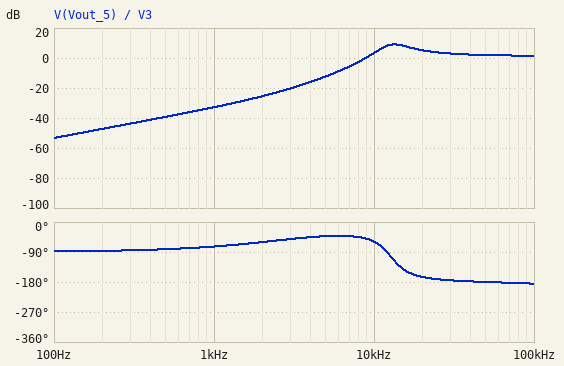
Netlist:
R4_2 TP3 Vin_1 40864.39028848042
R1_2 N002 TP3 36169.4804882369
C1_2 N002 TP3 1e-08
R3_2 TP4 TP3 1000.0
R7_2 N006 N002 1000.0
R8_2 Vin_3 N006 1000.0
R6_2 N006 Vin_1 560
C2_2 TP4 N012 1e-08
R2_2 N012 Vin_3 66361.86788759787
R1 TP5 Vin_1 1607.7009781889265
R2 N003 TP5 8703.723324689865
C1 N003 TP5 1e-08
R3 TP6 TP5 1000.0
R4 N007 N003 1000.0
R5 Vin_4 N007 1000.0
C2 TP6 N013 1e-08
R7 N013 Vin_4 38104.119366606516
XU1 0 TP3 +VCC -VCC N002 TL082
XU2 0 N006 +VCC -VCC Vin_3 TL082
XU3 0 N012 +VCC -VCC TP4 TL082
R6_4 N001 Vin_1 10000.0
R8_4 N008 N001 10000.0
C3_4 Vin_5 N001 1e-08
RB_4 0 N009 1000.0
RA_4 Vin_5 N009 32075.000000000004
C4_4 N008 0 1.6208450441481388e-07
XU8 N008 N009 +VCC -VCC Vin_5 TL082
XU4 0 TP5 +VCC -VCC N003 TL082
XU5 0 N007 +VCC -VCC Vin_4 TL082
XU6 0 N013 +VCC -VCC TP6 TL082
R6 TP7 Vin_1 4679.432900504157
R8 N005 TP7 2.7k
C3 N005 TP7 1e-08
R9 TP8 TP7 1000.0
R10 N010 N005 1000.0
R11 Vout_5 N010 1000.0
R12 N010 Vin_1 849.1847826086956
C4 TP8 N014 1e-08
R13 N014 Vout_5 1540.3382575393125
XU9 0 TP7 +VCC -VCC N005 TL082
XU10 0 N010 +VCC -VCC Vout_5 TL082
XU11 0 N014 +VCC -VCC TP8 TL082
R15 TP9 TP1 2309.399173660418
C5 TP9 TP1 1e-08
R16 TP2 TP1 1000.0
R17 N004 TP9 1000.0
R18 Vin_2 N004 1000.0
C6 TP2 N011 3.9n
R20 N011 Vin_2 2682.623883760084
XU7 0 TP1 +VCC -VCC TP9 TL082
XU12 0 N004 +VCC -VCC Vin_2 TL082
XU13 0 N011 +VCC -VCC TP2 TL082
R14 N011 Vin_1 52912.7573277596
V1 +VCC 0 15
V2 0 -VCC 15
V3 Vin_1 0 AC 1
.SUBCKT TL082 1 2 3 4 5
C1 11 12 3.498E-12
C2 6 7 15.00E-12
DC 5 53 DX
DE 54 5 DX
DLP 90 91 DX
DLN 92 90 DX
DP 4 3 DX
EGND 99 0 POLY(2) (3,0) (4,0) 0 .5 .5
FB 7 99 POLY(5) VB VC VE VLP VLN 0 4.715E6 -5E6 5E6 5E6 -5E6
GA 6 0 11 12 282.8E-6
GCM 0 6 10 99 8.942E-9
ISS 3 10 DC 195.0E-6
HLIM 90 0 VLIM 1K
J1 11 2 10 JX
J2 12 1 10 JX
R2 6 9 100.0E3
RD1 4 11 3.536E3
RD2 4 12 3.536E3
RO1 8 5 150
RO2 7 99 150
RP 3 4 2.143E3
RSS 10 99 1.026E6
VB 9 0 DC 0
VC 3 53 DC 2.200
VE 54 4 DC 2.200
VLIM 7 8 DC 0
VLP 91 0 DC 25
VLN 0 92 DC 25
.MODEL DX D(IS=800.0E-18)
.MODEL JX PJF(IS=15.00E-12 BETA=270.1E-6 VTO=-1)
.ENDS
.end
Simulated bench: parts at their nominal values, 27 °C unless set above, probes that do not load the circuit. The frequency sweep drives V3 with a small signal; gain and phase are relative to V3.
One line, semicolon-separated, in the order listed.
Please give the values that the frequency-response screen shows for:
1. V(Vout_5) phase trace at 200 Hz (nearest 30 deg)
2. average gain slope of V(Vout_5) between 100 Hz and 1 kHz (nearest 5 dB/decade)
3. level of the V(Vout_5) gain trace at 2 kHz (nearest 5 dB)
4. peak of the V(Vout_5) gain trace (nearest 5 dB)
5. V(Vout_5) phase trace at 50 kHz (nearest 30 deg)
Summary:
-90 deg; 20 dB/decade; -25 dB; 10 dB; -180 deg
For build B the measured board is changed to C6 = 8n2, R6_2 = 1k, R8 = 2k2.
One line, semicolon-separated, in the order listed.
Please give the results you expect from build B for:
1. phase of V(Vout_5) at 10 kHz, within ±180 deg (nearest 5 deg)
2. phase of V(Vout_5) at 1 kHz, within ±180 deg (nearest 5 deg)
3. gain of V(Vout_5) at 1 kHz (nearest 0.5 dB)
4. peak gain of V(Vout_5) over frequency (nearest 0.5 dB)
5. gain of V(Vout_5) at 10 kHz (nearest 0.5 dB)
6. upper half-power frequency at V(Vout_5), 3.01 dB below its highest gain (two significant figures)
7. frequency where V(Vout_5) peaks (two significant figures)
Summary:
-70 deg; -80 deg; -30.0 dB; 7.5 dB; 3.0 dB; 21 kHz; 14 kHz
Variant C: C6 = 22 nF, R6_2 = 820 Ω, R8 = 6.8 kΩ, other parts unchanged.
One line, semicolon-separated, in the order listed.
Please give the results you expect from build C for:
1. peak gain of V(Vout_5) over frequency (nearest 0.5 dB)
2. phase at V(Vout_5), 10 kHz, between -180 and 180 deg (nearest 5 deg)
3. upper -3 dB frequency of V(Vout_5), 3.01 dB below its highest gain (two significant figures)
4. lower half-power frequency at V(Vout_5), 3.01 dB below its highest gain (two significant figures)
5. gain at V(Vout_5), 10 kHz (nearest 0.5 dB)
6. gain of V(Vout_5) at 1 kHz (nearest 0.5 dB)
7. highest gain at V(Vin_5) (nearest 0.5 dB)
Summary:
17.5 dB; -15 deg; 14 kHz; 12 kHz; 5.0 dB; -41.5 dB; 52.0 dB
